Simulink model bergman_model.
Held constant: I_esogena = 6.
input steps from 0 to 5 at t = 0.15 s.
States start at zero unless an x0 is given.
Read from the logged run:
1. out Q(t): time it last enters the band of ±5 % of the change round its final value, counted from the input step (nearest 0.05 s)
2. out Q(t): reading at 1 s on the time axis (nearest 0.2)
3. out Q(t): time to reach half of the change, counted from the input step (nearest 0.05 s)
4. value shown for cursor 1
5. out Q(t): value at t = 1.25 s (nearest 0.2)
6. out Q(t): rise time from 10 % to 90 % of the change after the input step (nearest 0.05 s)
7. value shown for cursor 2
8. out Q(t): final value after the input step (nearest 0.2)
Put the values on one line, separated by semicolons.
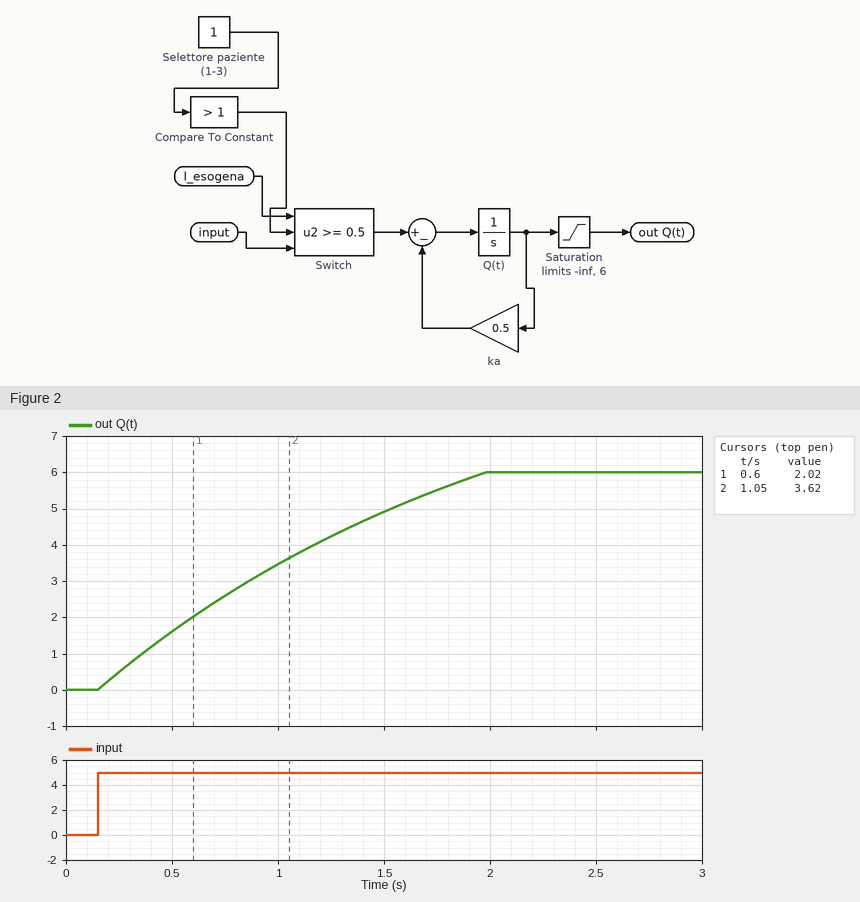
1.70 s; 3.4; 0.70 s; 2.02; 4.2; 1.45 s; 3.62; 6.0
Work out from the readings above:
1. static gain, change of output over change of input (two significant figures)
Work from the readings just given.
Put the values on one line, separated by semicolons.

1.2
